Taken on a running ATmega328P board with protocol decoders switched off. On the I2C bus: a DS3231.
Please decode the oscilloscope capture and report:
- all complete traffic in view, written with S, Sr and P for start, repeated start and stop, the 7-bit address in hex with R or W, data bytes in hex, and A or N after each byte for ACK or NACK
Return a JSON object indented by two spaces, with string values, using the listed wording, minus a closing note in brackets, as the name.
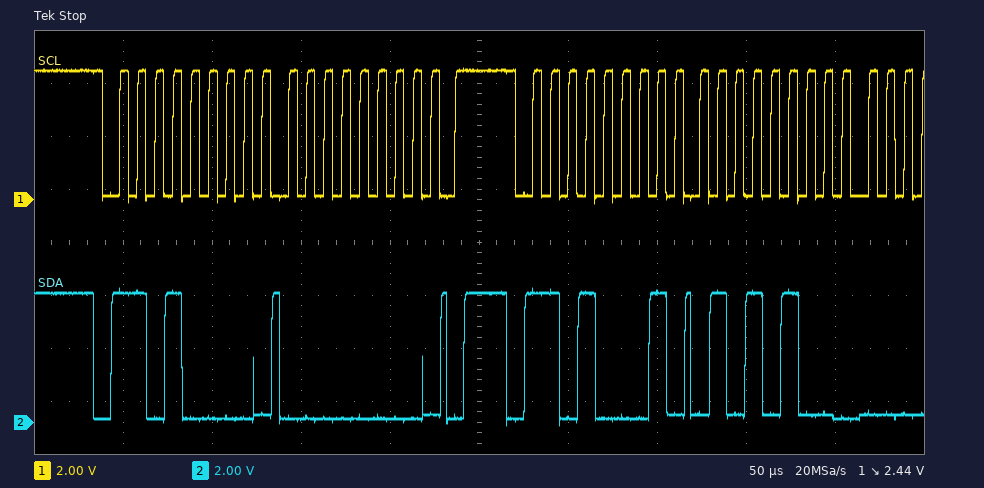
{
  "all complete traffic in view, written with S, Sr and P for start, repeated start and stop, the 7-bit address in hex with R or W, data bytes in hex, and A or N after each byte for ACK or NACK": "S 68W A 00 A P S 68R A 54 A"
}
